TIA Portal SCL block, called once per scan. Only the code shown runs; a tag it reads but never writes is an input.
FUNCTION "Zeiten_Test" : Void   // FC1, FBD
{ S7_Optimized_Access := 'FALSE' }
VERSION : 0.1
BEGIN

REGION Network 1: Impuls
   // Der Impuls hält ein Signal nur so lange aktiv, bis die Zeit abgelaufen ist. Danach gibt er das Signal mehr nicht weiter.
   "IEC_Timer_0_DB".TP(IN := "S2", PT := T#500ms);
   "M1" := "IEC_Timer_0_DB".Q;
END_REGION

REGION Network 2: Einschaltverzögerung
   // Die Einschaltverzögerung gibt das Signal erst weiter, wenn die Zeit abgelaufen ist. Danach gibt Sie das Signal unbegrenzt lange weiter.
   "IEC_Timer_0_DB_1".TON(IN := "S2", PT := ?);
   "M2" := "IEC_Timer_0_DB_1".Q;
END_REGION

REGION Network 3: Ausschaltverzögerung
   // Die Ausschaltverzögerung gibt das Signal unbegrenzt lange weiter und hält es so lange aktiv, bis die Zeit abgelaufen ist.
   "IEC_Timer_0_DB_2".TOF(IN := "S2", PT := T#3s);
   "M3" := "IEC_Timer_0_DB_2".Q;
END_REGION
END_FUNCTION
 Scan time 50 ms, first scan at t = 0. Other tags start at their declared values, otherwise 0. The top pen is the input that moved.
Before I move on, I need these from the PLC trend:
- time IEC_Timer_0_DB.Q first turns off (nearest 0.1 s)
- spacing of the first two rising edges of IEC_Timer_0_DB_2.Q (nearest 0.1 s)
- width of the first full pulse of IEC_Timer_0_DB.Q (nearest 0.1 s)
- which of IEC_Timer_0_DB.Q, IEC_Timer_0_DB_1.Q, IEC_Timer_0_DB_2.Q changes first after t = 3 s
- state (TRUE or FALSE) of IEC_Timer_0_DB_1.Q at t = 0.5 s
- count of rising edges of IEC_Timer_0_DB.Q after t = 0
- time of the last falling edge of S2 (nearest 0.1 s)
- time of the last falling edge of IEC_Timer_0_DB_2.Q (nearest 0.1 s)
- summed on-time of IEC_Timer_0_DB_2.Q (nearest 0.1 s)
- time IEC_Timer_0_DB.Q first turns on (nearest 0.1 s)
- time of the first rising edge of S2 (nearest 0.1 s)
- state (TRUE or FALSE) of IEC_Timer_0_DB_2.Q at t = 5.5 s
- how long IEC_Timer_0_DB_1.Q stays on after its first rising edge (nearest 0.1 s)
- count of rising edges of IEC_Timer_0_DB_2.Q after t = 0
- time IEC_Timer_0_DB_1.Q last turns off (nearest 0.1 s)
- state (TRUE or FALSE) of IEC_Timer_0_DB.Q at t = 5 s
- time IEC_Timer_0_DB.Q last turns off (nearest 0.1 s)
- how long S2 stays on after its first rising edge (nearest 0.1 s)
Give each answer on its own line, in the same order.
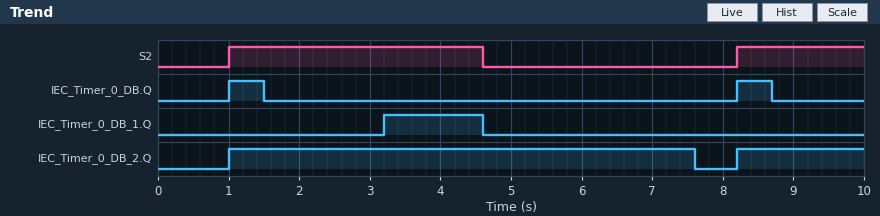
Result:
1.5 s
7.2 s
0.5 s
IEC_Timer_0_DB_1.Q
FALSE
2
4.6 s
7.6 s
8.4 s
1.0 s
1.0 s
TRUE
1.4 s
2
4.6 s
FALSE
8.7 s
3.6 s
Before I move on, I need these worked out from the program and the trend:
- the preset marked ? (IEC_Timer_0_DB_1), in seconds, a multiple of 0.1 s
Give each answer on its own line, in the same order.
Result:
2.2 s
